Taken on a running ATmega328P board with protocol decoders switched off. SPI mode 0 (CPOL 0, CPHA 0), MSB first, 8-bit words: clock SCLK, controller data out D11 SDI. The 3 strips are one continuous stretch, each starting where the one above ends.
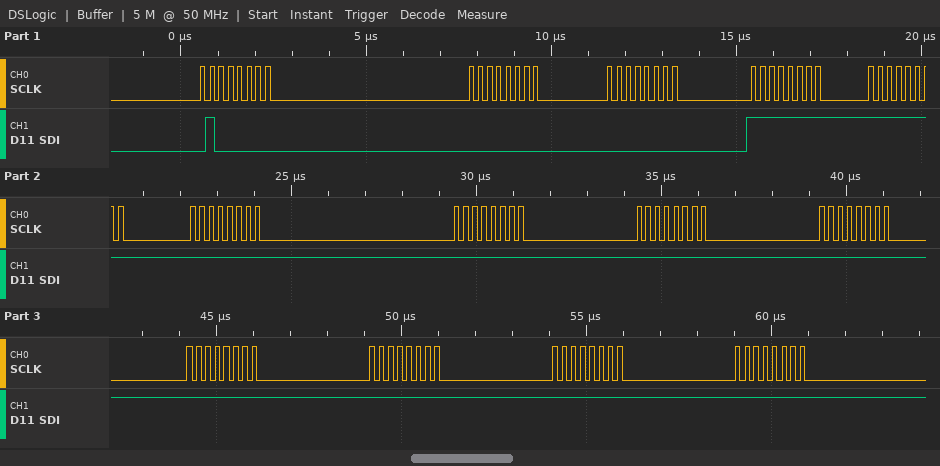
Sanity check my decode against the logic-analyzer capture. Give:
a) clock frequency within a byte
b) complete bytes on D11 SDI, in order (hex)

4 MHz
0x40 0x00 0x00 0xFF 0xFF 0xFF 0xFF 0xFF 0xFF 0xFF 0xFF 0xFF 0xFF
